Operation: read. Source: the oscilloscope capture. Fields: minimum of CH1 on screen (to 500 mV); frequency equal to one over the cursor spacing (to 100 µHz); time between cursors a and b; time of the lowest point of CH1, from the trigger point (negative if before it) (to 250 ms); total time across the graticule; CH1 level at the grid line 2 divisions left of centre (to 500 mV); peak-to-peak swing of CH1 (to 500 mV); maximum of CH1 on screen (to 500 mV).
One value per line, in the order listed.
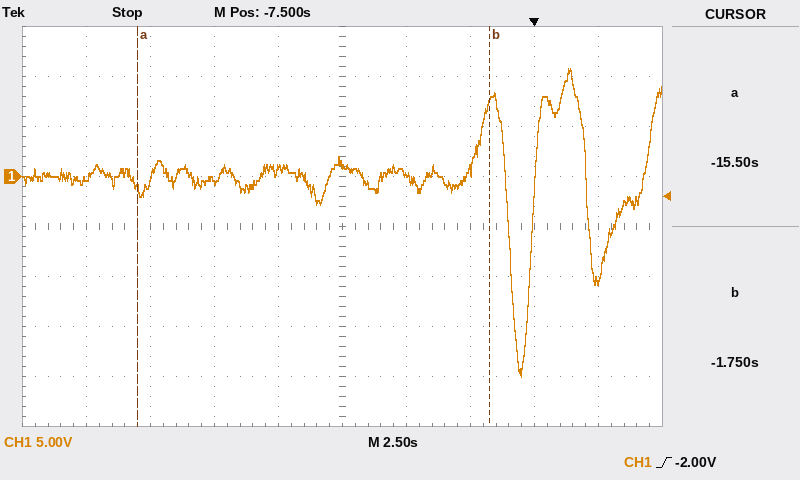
-20.0 V
72.7 mHz
13.75 s
-500 ms
25 s
-500 mV
31.0 V
11.0 V
